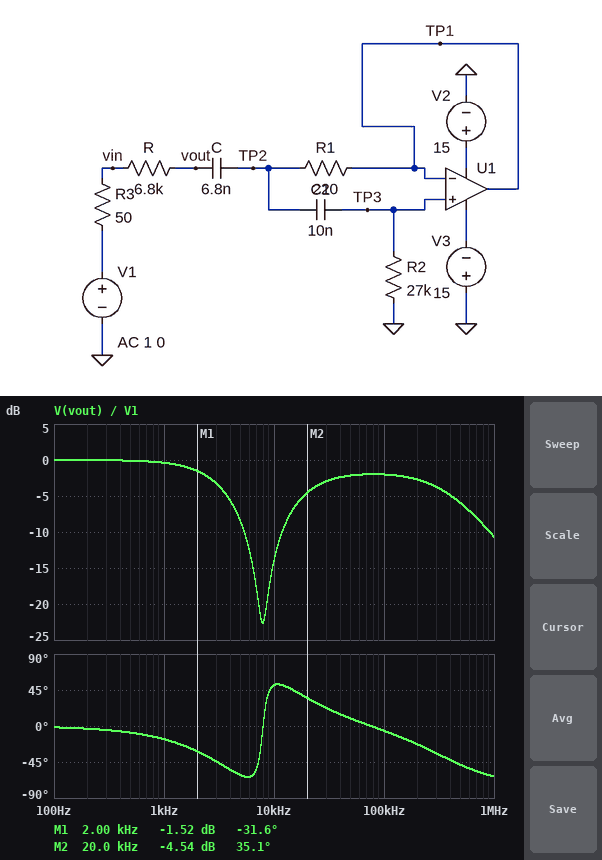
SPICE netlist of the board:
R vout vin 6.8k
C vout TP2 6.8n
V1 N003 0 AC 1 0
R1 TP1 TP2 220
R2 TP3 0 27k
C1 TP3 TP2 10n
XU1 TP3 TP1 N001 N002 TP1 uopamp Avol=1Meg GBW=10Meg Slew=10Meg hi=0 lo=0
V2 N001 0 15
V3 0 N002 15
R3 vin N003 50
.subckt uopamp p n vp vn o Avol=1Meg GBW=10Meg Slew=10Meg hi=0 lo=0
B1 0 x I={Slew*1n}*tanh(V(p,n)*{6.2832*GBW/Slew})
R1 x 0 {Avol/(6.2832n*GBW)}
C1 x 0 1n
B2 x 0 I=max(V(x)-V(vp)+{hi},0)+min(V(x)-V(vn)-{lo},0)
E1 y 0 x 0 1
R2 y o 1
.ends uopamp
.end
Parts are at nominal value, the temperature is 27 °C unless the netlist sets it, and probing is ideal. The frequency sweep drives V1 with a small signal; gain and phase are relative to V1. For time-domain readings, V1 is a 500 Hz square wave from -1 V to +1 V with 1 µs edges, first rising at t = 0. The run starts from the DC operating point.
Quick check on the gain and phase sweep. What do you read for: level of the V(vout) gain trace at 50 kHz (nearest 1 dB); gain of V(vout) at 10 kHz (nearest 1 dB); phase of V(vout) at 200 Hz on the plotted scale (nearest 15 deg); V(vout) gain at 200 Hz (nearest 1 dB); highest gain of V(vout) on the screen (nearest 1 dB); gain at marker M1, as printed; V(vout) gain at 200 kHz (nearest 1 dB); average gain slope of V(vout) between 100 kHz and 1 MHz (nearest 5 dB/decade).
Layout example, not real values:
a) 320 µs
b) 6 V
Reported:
a) -2 dB
b) -14 dB
c) 0 deg
d) 0 dB
e) 0 dB
f) -1.52 dB
g) -3 dB
h) -10 dB/decade
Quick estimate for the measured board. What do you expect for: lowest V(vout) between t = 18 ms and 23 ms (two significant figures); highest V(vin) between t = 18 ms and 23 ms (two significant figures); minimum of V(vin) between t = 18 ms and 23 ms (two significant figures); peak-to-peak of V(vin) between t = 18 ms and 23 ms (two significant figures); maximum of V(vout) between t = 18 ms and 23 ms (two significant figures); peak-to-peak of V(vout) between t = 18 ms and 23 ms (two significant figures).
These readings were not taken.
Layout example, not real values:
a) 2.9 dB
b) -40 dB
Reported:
a) -1.0 V
b) 1.0 V
c) -1.0 V
d) 2.0 V
e) 1.0 V
f) 2.0 V
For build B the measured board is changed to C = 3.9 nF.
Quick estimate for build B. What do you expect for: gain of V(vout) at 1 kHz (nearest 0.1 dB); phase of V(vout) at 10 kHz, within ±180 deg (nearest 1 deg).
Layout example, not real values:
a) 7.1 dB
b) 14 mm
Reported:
a) -0.1 dB
b) -25 deg
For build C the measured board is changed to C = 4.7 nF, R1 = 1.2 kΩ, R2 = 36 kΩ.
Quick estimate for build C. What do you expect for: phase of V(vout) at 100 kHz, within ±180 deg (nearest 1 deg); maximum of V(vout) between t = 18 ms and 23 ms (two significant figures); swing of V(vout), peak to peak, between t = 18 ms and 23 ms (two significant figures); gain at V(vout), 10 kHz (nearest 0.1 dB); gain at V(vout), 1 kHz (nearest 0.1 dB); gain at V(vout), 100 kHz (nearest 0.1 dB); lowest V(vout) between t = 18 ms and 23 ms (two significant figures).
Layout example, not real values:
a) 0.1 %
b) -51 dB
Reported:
a) -2 deg
b) 1.1 V
c) 2.2 V
d) -2.1 dB
e) -0.3 dB
f) -1.5 dB
g) -1.1 V
